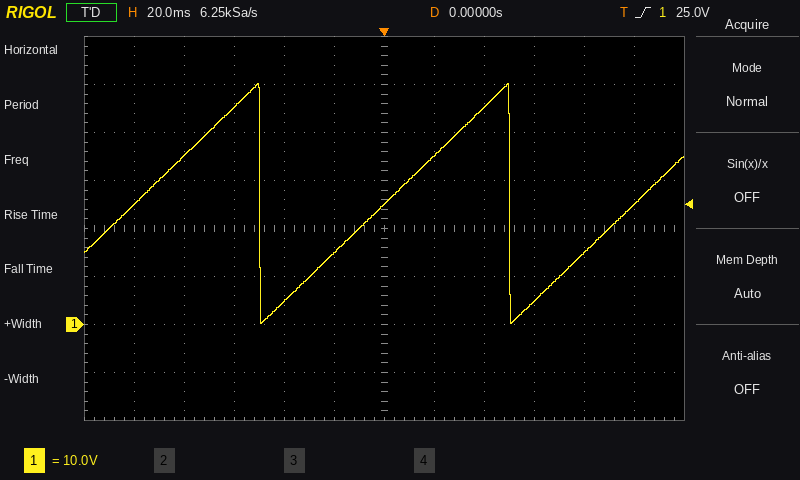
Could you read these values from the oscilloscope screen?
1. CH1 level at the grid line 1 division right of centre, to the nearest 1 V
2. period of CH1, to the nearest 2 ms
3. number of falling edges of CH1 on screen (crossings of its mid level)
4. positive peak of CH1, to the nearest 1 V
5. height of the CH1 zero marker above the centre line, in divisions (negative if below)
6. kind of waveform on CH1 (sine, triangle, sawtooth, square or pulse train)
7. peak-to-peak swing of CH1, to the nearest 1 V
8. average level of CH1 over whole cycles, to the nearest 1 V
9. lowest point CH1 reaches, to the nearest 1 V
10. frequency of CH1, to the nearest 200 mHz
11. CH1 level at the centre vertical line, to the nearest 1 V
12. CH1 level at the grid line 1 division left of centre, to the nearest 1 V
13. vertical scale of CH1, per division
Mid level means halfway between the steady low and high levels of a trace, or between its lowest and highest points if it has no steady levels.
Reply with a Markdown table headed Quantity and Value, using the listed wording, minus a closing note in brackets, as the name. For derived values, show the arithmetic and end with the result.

| Quantity | Value |
|---|---|
| CH1 level at the grid line 1 division right of centre, to the nearest 1 V | 35 V |
| period of CH1, to the nearest 2 ms | 100 ms |
| number of falling edges of CH1 on screen | 2 |
| positive peak of CH1, to the nearest 1 V | 50 V |
| height of the CH1 zero marker above the centre line, in divisions | -2.0 div |
| kind of waveform on CH1 | sawtooth |
| peak-to-peak swing of CH1, to the nearest 1 V | 50 V − (0 V) = 50 V |
| average level of CH1 over whole cycles, to the nearest 1 V | (50 V + (0 V)) / 2 ≈ 25 V |
| lowest point CH1 reaches, to the nearest 1 V | 0 V |
| frequency of CH1, to the nearest 200 mHz | 1 / 100 ms ≈ 10.0 Hz |
| CH1 level at the centre vertical line, to the nearest 1 V | 25 V |
| CH1 level at the grid line 1 division left of centre, to the nearest 1 V | 15 V |
| vertical scale of CH1, per division | 10 V |
